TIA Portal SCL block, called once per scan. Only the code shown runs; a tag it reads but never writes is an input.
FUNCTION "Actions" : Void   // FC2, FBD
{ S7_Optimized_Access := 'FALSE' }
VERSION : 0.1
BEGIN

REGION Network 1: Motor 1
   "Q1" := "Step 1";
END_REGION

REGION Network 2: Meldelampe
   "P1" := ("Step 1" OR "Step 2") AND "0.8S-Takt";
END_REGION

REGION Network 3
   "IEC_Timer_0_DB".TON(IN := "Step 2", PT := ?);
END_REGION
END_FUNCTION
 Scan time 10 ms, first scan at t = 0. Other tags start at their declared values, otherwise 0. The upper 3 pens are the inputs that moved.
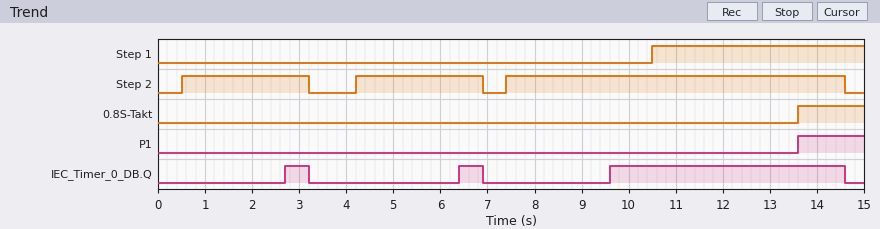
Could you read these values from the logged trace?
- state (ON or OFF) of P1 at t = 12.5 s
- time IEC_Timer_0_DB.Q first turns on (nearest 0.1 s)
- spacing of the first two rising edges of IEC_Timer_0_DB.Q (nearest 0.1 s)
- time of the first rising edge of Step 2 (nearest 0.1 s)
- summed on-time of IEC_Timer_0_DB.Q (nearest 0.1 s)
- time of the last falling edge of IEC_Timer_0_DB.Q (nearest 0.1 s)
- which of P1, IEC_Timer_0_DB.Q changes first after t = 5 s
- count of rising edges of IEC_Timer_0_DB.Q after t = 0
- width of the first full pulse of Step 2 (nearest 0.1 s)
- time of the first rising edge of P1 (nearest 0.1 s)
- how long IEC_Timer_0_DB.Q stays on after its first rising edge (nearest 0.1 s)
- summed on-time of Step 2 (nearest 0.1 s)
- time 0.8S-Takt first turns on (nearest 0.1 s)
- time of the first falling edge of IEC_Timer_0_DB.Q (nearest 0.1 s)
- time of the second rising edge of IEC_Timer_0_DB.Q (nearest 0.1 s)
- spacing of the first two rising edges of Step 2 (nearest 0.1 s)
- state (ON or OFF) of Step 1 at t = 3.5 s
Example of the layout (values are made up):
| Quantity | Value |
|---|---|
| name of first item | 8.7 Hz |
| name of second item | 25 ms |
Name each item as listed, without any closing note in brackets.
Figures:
| Quantity | Value |
|---|---|
| state (ON or OFF) of P1 at t = 12.5 s | OFF |
| time IEC_Timer_0_DB.Q first turns on | 2.7 s |
| spacing of the first two rising edges of IEC_Timer_0_DB.Q | 3.7 s |
| time of the first rising edge of Step 2 | 0.5 s |
| summed on-time of IEC_Timer_0_DB.Q | 6.0 s |
| time of the last falling edge of IEC_Timer_0_DB.Q | 14.6 s |
| which of P1, IEC_Timer_0_DB.Q changes first after t = 5 s | IEC_Timer_0_DB.Q |
| count of rising edges of IEC_Timer_0_DB.Q after t = 0 | 3 |
| width of the first full pulse of Step 2 | 2.7 s |
| time of the first rising edge of P1 | 13.6 s |
| how long IEC_Timer_0_DB.Q stays on after its first rising edge | 0.5 s |
| summed on-time of Step 2 | 12.6 s |
| time 0.8S-Takt first turns on | 13.6 s |
| time of the first falling edge of IEC_Timer_0_DB.Q | 3.2 s |
| time of the second rising edge of IEC_Timer_0_DB.Q | 6.4 s |
| spacing of the first two rising edges of Step 2 | 3.7 s |
| state (ON or OFF) of Step 1 at t = 3.5 s | OFF |
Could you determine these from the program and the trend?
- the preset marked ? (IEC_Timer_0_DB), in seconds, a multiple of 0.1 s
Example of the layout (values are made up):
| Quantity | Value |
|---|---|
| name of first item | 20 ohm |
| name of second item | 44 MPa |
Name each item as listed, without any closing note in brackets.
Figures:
| Quantity | Value |
|---|---|
| the preset marked ? (IEC_Timer_0_DB), in seconds, a multiple of 0.1 s | 2.2 s |
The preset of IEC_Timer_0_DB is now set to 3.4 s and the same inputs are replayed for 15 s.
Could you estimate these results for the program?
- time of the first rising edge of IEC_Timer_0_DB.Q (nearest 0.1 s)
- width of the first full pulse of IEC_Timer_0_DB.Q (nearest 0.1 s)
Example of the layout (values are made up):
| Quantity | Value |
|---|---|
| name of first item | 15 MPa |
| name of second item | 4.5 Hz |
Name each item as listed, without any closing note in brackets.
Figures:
| Quantity | Value |
|---|---|
| time of the first rising edge of IEC_Timer_0_DB.Q | 10.8 s |
| width of the first full pulse of IEC_Timer_0_DB.Q | 3.8 s |
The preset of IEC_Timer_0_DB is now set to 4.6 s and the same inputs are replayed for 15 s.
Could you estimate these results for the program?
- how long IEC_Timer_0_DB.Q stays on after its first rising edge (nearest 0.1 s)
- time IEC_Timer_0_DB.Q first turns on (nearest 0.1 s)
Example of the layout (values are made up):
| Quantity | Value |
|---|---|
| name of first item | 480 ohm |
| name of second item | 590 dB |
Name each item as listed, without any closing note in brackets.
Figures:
| Quantity | Value |
|---|---|
| how long IEC_Timer_0_DB.Q stays on after its first rising edge | 2.6 s |
| time IEC_Timer_0_DB.Q first turns on | 12.0 s |
